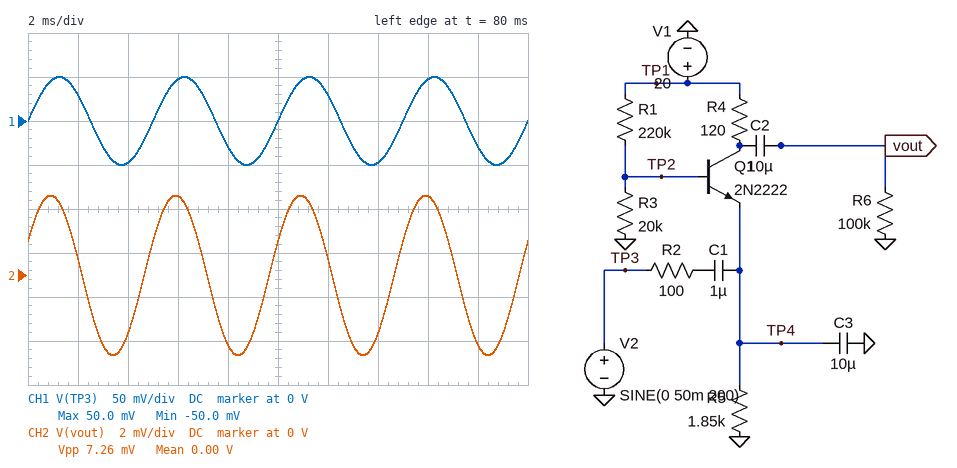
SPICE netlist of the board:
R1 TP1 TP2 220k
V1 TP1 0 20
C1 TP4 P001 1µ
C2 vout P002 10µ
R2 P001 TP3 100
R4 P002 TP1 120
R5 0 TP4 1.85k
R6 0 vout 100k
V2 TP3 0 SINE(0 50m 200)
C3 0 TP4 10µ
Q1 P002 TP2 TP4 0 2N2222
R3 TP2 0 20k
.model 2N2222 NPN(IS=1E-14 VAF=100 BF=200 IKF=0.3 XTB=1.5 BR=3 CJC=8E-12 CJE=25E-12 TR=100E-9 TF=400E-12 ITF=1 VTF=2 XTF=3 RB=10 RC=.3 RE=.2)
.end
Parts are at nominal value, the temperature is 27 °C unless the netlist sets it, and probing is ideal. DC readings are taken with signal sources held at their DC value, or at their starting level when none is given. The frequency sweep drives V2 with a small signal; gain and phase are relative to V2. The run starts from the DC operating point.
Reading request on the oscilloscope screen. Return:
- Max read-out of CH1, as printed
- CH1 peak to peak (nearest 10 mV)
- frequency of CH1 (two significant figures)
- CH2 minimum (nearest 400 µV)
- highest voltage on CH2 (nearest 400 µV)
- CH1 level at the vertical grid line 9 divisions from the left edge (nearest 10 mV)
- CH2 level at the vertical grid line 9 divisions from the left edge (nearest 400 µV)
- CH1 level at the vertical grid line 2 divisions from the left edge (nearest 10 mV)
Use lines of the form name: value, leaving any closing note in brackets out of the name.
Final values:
Max read-out of CH1, as printed: 50.0 mV
CH1 peak to peak: 100 mV
frequency of CH1: 200 Hz
CH2 minimum: -3.6 mV
highest voltage on CH2: 3.6 mV
CH1 level at the vertical grid line 9 divisions from the left edge: -30 mV
CH2 level at the vertical grid line 9 divisions from the left edge: -3.2 mV
CH1 level at the vertical grid line 2 divisions from the left edge: -50 mV
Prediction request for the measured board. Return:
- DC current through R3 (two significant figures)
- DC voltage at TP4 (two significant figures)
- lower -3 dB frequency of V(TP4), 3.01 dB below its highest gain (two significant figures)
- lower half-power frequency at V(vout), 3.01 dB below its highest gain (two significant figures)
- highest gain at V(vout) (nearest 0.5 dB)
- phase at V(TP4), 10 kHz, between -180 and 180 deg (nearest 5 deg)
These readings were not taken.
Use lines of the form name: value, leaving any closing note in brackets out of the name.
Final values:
DC current through R3: 81 µA
DC voltage at TP4: 990 mV
lower -3 dB frequency of V(TP4), 3.01 dB below its highest gain: 110 Hz
lower half-power frequency at V(vout), 3.01 dB below its highest gain: 110 Hz
highest gain at V(vout): -22.0 dB
phase at V(TP4), 10 kHz, between -180 and 180 deg: -80 deg
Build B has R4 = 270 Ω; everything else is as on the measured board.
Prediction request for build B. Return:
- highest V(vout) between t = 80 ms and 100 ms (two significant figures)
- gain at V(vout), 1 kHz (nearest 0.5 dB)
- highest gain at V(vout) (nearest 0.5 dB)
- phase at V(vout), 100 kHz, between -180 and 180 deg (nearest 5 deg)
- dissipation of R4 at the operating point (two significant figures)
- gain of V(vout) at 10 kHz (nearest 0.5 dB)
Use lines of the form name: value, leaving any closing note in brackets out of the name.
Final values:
highest V(vout) between t = 80 ms and 100 ms: 8.1 mV
gain at V(vout), 1 kHz: -15.5 dB
highest gain at V(vout): -15.0 dB
phase at V(vout), 100 kHz, between -180 and 180 deg: -105 deg
dissipation of R4 at the operating point: 77 µW
gain of V(vout) at 10 kHz: -29.5 dB
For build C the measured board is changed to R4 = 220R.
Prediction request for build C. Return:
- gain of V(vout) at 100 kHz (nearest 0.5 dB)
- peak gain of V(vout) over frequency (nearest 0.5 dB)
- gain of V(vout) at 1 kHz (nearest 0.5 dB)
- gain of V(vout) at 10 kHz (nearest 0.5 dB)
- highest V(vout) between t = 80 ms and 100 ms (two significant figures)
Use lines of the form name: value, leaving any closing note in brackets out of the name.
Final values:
gain of V(vout) at 100 kHz: -51.5 dB
peak gain of V(vout) over frequency: -16.5 dB
gain of V(vout) at 1 kHz: -17.5 dB
gain of V(vout) at 10 kHz: -31.5 dB
highest V(vout) between t = 80 ms and 100 ms: 6.6 mV
